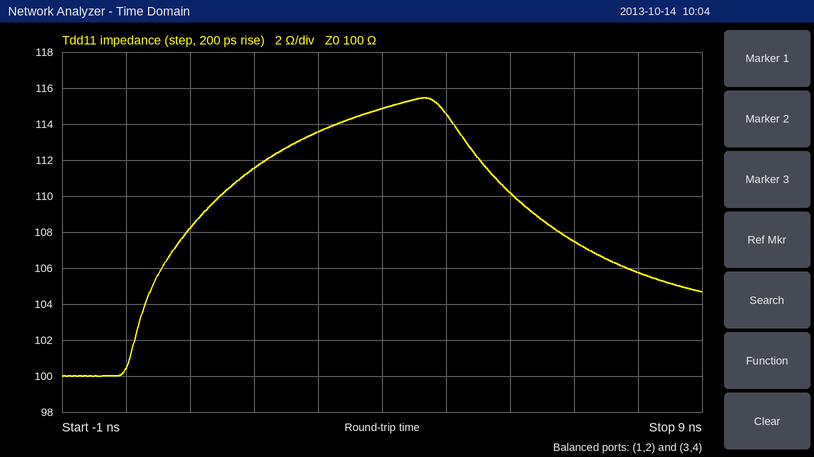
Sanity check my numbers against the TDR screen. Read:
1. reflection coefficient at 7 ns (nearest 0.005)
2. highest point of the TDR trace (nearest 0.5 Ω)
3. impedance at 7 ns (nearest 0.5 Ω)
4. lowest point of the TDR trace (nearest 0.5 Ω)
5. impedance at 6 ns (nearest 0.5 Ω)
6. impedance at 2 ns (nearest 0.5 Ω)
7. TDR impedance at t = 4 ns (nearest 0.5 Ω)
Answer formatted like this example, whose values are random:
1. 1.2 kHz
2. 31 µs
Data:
1. +0.035
2. 115.5 Ω
3. 107.5 Ω
4. 100.0 Ω
5. 110.0 Ω
6. 111.5 Ω
7. 115.0 Ω
